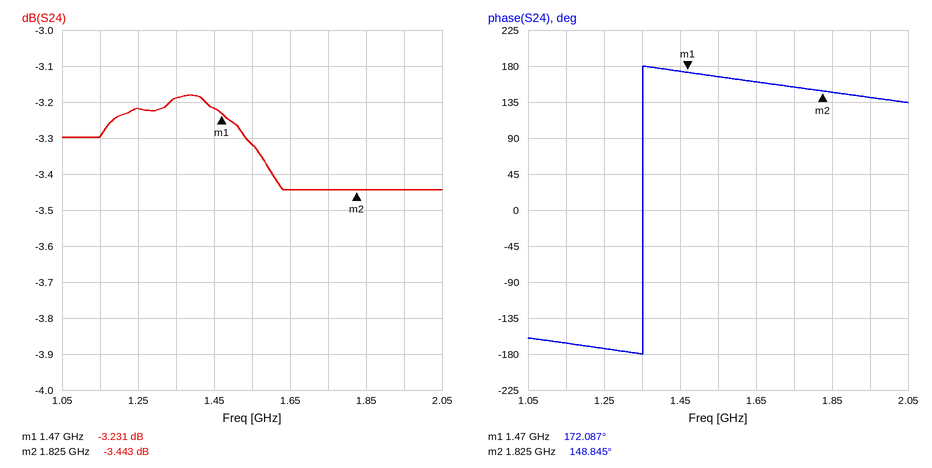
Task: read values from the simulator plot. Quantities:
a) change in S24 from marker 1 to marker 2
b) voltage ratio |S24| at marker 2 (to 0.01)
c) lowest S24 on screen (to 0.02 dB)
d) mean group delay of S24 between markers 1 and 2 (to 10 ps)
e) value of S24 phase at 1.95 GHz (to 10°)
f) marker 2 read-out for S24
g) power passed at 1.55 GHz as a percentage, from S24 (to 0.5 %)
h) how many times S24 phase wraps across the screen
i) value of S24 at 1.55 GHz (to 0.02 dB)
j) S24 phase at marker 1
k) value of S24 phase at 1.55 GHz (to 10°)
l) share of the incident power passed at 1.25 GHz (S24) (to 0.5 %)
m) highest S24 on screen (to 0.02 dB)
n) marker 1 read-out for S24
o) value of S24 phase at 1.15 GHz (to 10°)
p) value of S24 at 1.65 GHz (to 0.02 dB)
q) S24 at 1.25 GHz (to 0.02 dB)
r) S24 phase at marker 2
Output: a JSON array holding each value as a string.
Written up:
["-0.212 dB", "0.67", "-3.44 dB", "180 ps", "140°", "-3.443 dB", "46.5 %", "1", "-3.32 dB", "172.087°", "170°", "47.5 %", "-3.18 dB", "-3.231 dB", "-170°", "-3.44 dB", "-3.22 dB", "148.845°"]
